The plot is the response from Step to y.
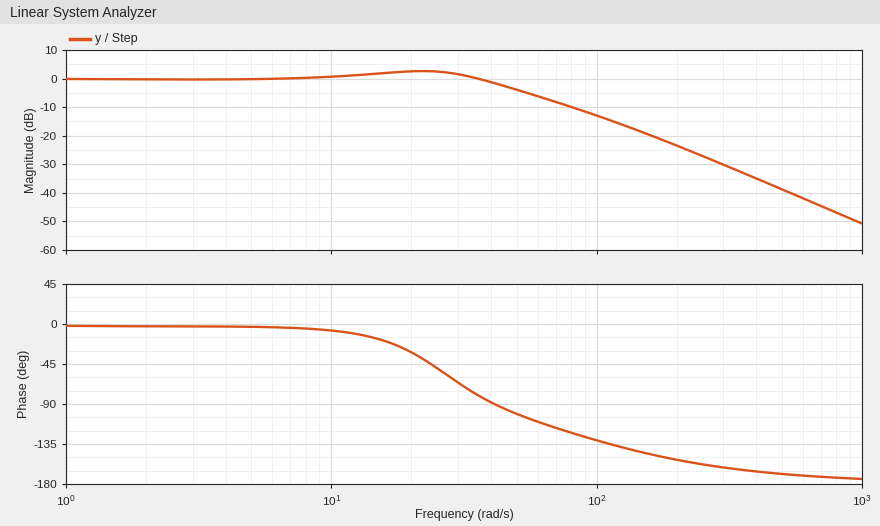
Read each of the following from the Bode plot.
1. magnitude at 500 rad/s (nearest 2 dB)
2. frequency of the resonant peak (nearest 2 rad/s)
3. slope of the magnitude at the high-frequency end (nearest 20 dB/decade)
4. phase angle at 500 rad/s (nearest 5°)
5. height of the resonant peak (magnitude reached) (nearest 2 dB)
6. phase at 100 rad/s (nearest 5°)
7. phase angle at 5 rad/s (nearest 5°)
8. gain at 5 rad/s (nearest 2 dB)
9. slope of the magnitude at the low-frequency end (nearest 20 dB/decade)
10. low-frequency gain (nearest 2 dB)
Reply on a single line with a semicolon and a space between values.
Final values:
-38 dB; 22 rad/s; -40 dB/decade; -170°; 2 dB; -130°; -5°; 0 dB; 0 dB/decade; 0 dB
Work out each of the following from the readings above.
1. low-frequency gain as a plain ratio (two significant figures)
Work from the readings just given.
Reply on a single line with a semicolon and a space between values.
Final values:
1.0
